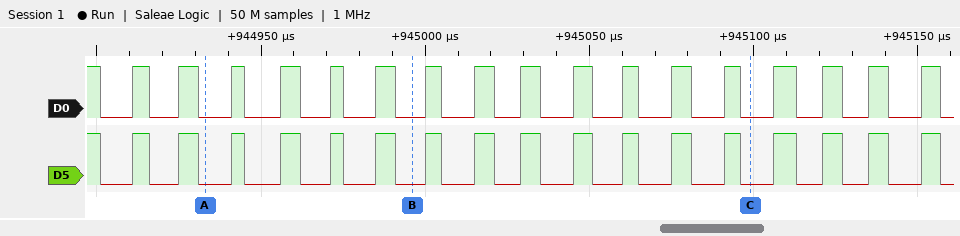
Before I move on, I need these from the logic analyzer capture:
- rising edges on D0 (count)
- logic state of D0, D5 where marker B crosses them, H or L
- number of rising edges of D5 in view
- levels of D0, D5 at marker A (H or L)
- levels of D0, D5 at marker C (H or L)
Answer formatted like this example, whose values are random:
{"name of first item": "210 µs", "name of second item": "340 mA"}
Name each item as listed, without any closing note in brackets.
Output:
{"rising edges on D0": "17", "logic state of D0, D5 where marker B crosses them, H or L": "D0=L, D5=L", "number of rising edges of D5 in view": "17", "levels of D0, D5 at marker A": "D0=L, D5=L", "levels of D0, D5 at marker C": "D0=L, D5=L"}
